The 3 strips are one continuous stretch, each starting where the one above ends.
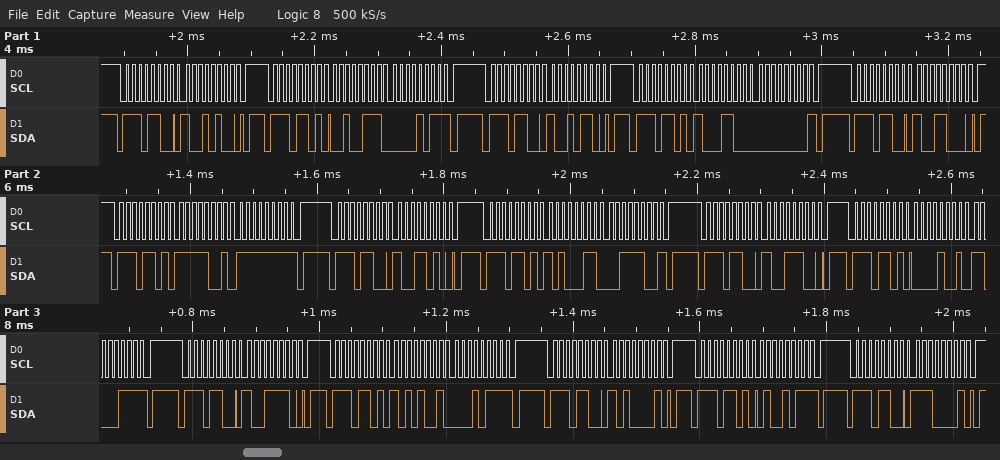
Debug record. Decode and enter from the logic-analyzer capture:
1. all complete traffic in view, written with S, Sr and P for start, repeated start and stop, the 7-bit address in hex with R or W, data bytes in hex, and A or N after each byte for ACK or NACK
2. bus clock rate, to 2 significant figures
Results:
S 76W A 94 A P S 76R A 27 A 0B N P S 76W A 96 A P S 76R A 8C A 00 N P S 76W A 98 A P S 76R A F9 A FF N P S 76W A 9A A P S 76R A A3 A 3C N P S 76W A 9C A P S 76R A 09 A C7 N P S 76W A 9E A P S 76R A A9 A 17 N P S 76W A A1 A P S 76R A 4B N P S 76W A E1 A P
100 kHz
